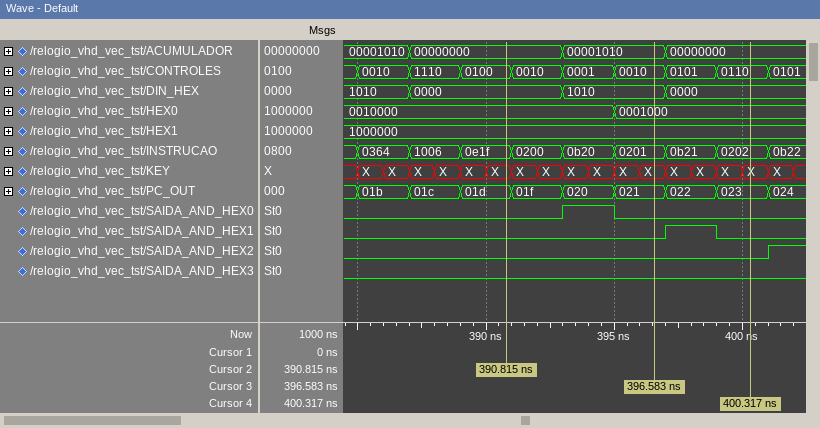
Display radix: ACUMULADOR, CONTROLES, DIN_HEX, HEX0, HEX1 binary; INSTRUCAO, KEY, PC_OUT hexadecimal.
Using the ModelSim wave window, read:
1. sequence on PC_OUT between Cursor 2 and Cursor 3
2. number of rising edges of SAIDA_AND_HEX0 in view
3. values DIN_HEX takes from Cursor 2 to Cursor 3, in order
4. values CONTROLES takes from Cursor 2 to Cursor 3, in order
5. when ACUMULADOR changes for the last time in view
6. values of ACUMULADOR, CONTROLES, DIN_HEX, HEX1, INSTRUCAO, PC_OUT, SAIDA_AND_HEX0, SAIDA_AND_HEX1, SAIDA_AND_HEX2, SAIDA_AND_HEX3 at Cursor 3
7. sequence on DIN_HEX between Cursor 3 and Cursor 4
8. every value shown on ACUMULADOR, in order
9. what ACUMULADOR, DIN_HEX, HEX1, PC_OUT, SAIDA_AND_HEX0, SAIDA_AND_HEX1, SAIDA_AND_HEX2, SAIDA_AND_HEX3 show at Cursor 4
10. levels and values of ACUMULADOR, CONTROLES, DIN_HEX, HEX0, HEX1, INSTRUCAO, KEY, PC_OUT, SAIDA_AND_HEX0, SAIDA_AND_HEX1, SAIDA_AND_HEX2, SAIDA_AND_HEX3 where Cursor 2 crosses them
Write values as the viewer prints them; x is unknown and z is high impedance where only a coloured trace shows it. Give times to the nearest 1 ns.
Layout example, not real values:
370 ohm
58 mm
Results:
01d, 01f, 020, 021
1
0000, 1010
0100, 0010, 0001, 0010
397 ns
ACUMULADOR=00001010, CONTROLES=0010, DIN_HEX=1010, HEX1=1000000, INSTRUCAO=0201, PC_OUT=021, SAIDA_AND_HEX0=0, SAIDA_AND_HEX1=0, SAIDA_AND_HEX2=0, SAIDA_AND_HEX3=0
1010, 0000
00001010, 00000000, 00001010, 00000000
ACUMULADOR=00000000, DIN_HEX=0000, HEX1=1000000, PC_OUT=023, SAIDA_AND_HEX0=0, SAIDA_AND_HEX1=0, SAIDA_AND_HEX2=0, SAIDA_AND_HEX3=0
ACUMULADOR=00000000, CONTROLES=0100, DIN_HEX=0000, HEX0=0010000, HEX1=1000000, INSTRUCAO=0e1f, KEY=X, PC_OUT=01d, SAIDA_AND_HEX0=0, SAIDA_AND_HEX1=0, SAIDA_AND_HEX2=0, SAIDA_AND_HEX3=0
